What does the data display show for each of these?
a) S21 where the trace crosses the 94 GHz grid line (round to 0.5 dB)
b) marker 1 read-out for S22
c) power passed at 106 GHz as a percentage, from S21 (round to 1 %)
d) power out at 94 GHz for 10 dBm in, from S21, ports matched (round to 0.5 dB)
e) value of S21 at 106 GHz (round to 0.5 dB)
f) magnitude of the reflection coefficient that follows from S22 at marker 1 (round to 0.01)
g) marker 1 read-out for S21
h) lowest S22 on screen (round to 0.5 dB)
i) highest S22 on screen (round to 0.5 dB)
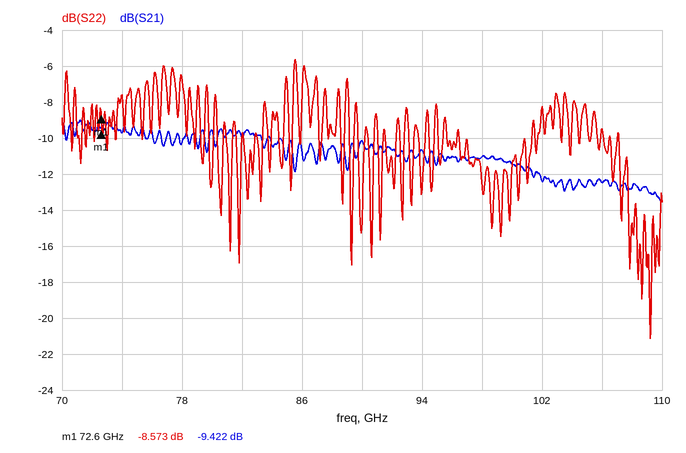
-10.5 dB
-8.573 dB
6 %
-0.5 dBm
-12.5 dB
0.37
-9.422 dB
-21.0 dB
-5.5 dB
